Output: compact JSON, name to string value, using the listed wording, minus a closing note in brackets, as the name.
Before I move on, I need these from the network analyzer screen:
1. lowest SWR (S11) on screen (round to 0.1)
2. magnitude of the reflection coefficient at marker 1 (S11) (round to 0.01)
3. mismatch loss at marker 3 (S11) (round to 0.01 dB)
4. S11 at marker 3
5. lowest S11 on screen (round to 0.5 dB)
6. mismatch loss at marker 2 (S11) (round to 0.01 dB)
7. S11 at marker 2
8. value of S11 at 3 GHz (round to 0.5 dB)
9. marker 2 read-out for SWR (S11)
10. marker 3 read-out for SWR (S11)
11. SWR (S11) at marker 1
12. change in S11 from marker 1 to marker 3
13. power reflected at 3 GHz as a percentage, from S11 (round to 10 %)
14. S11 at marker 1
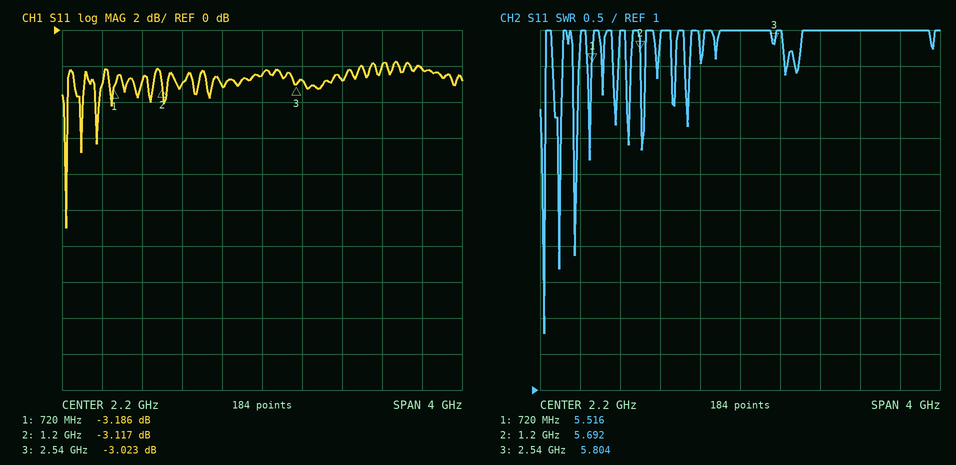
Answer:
{"lowest SWR (S11) on screen": "1.8", "magnitude of the reflection coefficient at marker 1 (S11)": "0.69", "mismatch loss at marker 3 (S11)": "3.00 dB", "S11 at marker 3": "-3.023 dB", "lowest S11 on screen": "-11.0 dB", "mismatch loss at marker 2 (S11)": "2.91 dB", "S11 at marker 2": "-3.117 dB", "value of S11 at 3 GHz": "-3.0 dB", "marker 2 read-out for SWR": "5.692", "marker 3 read-out for SWR": "5.804", "SWR (S11) at marker 1": "5.516", "change in S11 from marker 1 to marker 3": "0.163 dB", "power reflected at 3 GHz as a percentage, from S11": "50 %", "S11 at marker 1": "-3.186 dB"}
